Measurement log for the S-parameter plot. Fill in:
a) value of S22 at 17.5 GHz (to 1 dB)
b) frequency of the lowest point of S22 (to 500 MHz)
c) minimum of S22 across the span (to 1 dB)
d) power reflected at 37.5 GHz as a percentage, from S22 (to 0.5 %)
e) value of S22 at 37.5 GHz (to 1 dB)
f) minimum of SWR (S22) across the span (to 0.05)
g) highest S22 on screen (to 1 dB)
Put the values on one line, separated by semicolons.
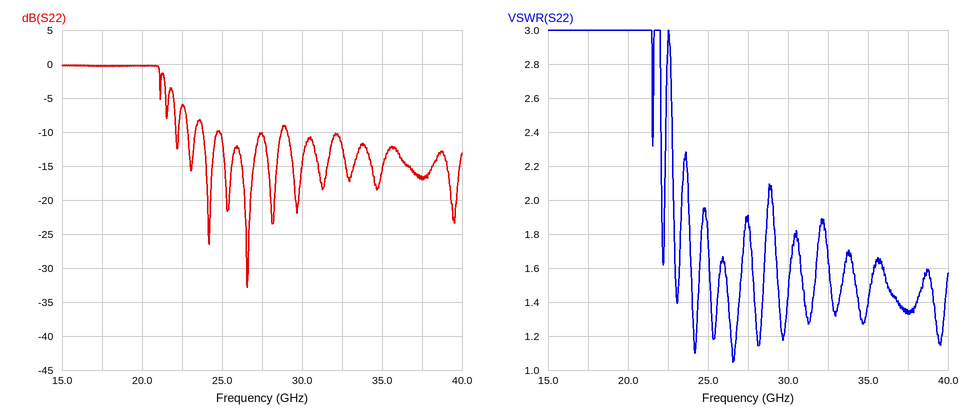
0 dB; 26.5 GHz; -33 dB; 2.0 %; -17 dB; 1.05; 0 dB
